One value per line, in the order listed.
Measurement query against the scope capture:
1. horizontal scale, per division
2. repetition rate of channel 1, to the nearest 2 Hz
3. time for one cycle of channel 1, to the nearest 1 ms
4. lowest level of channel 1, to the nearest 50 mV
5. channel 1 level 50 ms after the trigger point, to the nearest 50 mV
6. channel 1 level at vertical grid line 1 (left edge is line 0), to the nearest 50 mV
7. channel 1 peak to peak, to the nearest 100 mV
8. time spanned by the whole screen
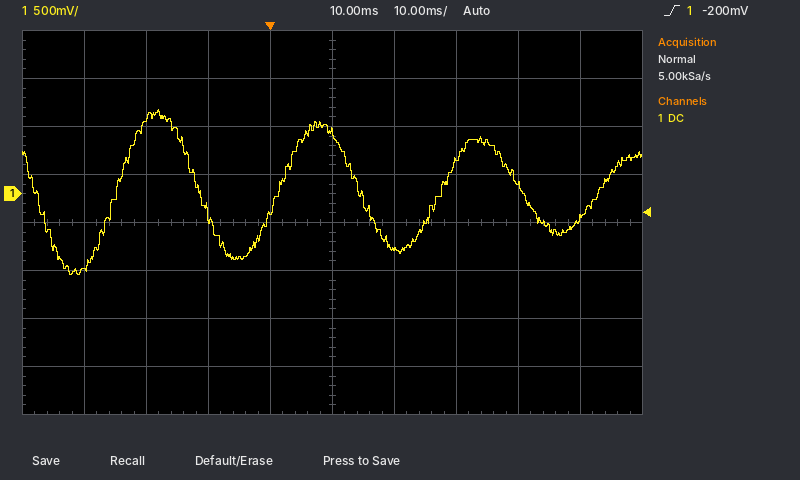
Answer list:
10 ms
38 Hz
26 ms
-850 mV
-250 mV
-800 mV
1.70 V
100 ms
